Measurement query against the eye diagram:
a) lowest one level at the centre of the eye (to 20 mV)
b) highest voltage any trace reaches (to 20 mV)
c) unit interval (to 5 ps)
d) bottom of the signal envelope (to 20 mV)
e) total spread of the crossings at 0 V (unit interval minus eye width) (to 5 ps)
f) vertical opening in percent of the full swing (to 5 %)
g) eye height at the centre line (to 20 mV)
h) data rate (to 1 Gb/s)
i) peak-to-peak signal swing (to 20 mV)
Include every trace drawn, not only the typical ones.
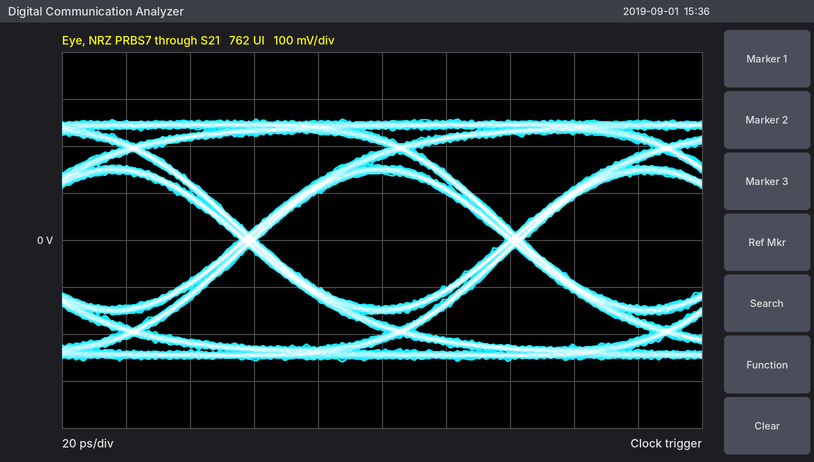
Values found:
140 mV
260 mV
85 ps
-260 mV
5 ps
55 %
280 mV
12 Gb/s
520 mV
